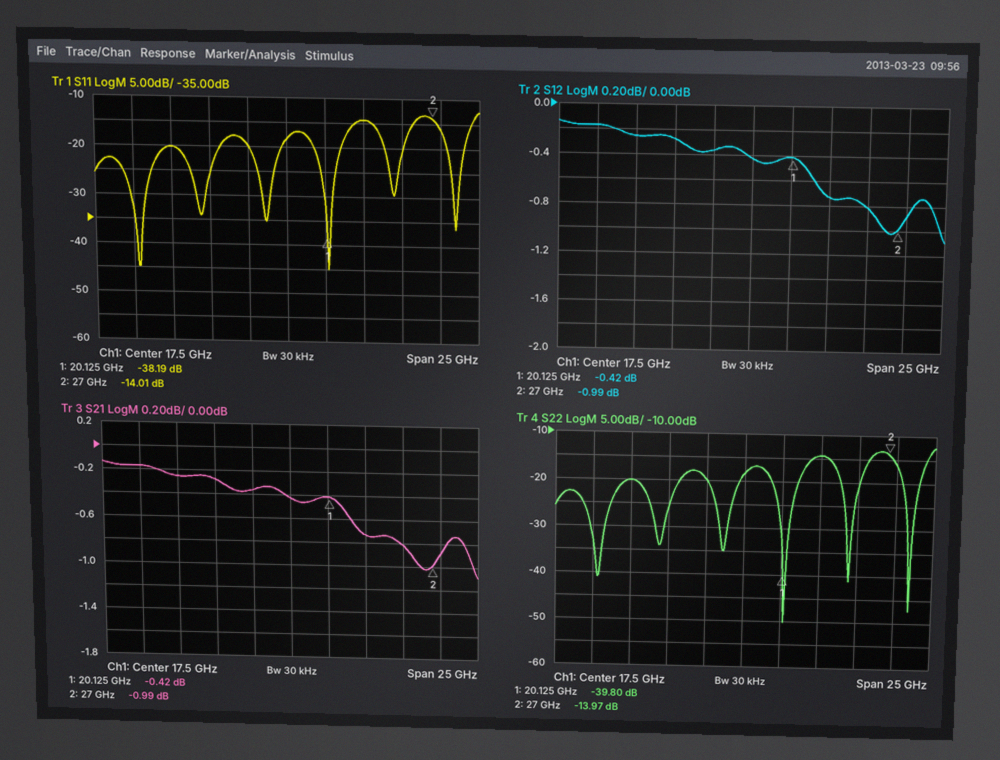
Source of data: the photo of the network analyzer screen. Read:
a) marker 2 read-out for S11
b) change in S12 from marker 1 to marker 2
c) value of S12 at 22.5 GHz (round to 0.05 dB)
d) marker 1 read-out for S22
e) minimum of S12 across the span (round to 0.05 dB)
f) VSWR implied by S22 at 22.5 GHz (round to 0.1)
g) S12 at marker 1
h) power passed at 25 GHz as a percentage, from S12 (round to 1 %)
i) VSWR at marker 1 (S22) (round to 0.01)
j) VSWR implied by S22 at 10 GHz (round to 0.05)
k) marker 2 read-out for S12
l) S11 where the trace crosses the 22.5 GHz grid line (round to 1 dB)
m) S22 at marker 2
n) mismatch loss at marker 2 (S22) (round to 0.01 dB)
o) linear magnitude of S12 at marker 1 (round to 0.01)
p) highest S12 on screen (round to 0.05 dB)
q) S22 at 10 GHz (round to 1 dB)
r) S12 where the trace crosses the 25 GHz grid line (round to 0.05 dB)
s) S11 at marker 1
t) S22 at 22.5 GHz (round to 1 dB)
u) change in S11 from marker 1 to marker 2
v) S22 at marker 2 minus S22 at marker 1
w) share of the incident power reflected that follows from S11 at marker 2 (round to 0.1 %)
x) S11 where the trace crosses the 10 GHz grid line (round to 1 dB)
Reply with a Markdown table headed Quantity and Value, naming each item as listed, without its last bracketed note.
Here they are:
| Quantity | Value |
|---|---|
| marker 2 read-out for S11 | -14.01 dB |
| change in S12 from marker 1 to marker 2 | -0.57 dB |
| value of S12 at 22.5 GHz | -0.75 dB |
| marker 1 read-out for S22 | -39.80 dB |
| minimum of S12 across the span | -1.10 dB |
| VSWR implied by S22 at 22.5 GHz | 1.5 |
| S12 at marker 1 | -0.42 dB |
| power passed at 25 GHz as a percentage, from S12 | 83 % |
| VSWR at marker 1 (S22) | 1.02 |
| VSWR implied by S22 at 10 GHz | 1.20 |
| marker 2 read-out for S12 | -0.99 dB |
| S11 where the trace crosses the 22.5 GHz grid line | -14 dB |
| S22 at marker 2 | -13.97 dB |
| mismatch loss at marker 2 (S22) | 0.18 dB |
| linear magnitude of S12 at marker 1 | 0.95 |
| highest S12 on screen | -0.15 dB |
| S22 at 10 GHz | -20 dB |
| S12 where the trace crosses the 25 GHz grid line | -0.80 dB |
| S11 at marker 1 | -38.19 dB |
| S22 at 22.5 GHz | -14 dB |
| change in S11 from marker 1 to marker 2 | 24.18 dB |
| S22 at marker 2 minus S22 at marker 1 | 25.83 dB |
| share of the incident power reflected that follows from S11 at marker 2 | 4.0 % |
| S11 where the trace crosses the 10 GHz grid line | -20 dB |
